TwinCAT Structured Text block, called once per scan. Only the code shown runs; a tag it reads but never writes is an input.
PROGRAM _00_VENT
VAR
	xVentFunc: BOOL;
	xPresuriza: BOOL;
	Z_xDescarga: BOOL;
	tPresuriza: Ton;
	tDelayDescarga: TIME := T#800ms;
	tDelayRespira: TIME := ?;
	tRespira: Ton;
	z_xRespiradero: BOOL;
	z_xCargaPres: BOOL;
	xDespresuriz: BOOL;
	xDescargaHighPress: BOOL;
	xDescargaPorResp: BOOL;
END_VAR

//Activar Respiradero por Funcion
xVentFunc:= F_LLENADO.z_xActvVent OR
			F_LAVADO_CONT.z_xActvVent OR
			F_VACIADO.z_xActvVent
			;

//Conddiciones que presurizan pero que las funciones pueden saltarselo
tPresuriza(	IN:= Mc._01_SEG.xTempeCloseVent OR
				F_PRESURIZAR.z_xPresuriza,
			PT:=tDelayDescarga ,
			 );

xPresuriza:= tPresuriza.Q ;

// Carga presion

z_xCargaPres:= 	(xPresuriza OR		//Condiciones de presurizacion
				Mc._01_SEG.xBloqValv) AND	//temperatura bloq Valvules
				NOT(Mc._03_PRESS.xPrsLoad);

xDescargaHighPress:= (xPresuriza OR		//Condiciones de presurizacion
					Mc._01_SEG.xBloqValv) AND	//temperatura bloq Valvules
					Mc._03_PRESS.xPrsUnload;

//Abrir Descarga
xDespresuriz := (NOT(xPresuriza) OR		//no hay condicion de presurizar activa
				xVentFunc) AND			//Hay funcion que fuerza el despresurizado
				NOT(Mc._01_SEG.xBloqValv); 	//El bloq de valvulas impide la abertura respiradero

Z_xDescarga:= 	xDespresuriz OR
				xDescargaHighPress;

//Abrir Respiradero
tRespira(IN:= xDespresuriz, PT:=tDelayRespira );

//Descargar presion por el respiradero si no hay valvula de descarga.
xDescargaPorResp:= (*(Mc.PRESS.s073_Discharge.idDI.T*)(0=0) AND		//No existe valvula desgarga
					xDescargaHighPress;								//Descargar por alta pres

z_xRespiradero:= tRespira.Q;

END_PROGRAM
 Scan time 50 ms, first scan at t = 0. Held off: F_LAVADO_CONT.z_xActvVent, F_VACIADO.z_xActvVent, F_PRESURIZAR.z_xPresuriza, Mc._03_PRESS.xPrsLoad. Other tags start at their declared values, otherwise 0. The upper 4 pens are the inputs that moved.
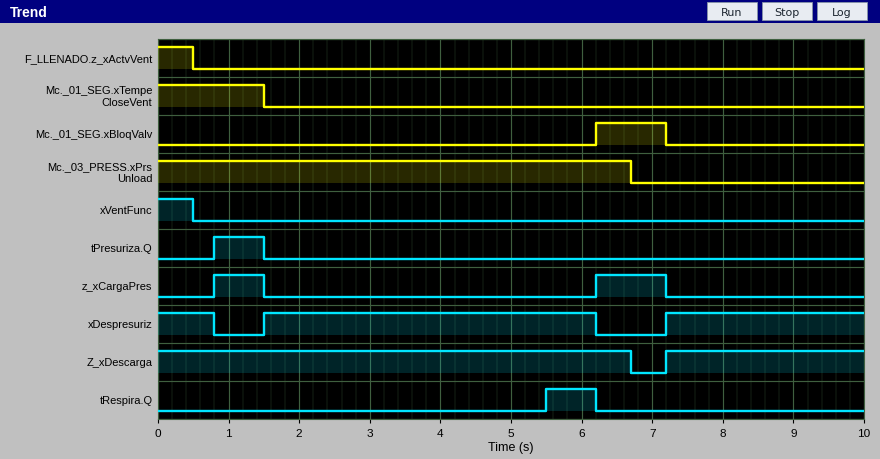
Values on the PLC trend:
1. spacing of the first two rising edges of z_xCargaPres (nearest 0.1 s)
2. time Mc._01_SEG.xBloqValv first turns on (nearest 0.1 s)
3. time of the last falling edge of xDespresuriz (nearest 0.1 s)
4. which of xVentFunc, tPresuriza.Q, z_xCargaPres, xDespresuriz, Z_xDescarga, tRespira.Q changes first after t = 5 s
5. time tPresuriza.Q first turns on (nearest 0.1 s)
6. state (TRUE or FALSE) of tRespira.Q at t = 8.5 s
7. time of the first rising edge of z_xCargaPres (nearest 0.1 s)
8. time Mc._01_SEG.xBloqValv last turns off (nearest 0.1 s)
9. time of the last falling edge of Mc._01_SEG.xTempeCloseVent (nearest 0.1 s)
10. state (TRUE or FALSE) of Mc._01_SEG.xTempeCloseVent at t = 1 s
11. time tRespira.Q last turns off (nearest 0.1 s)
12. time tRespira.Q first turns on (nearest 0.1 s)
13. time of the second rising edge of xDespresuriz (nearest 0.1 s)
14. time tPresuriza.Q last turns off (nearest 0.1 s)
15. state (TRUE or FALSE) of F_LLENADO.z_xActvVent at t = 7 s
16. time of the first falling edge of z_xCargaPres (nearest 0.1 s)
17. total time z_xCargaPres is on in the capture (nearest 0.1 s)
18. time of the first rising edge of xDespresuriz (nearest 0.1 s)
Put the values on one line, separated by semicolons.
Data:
5.4 s; 6.2 s; 6.2 s; tRespira.Q; 0.8 s; FALSE; 0.8 s; 7.2 s; 1.5 s; TRUE; 6.2 s; 5.5 s; 7.2 s; 1.5 s; FALSE; 1.5 s; 1.7 s; 1.5 s
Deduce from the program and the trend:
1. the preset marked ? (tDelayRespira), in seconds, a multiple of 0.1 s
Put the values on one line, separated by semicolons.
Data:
4.0 s
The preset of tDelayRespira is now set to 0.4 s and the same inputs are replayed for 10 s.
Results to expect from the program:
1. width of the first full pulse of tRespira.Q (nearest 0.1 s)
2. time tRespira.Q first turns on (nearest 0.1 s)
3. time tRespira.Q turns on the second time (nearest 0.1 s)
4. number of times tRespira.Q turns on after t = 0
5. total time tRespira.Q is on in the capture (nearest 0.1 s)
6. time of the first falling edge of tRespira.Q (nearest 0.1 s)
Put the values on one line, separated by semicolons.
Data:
0.4 s; 0.4 s; 1.9 s; 3; 7.1 s; 0.8 s
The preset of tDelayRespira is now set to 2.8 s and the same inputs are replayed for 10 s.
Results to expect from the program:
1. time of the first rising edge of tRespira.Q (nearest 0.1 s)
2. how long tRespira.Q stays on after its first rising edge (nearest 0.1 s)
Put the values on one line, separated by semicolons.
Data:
4.3 s; 1.9 s
